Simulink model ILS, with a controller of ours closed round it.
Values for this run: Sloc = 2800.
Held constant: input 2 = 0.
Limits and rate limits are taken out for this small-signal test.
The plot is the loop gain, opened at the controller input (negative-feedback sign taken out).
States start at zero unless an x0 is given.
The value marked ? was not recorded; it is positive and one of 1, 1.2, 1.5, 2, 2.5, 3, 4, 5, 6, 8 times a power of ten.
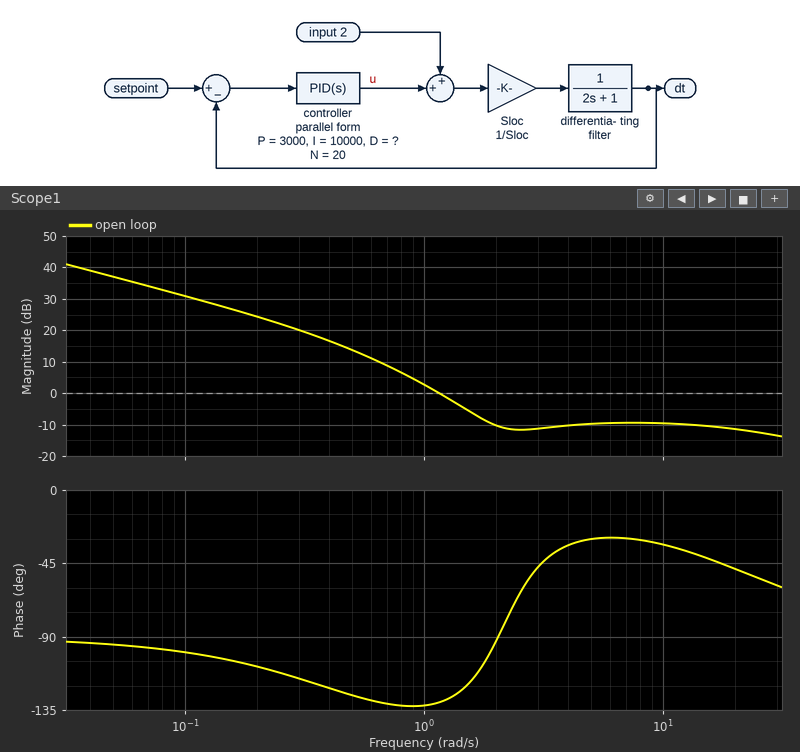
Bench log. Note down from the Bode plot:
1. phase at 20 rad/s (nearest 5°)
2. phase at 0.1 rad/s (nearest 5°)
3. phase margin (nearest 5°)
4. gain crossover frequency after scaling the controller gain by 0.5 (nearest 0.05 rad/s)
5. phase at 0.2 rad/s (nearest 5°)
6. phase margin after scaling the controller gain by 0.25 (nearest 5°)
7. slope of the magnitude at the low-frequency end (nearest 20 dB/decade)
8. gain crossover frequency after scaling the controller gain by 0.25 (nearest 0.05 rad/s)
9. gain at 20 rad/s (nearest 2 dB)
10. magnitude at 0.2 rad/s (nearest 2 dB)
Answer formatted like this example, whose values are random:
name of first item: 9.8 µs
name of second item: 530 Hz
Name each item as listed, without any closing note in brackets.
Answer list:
phase at 20 rad/s: -50°
phase at 0.1 rad/s: -100°
phase margin: 50°
gain crossover frequency after scaling the controller gain by 0.5: 0.85 rad/s
phase at 0.2 rad/s: -110°
phase margin after scaling the controller gain by 0.25: 50°
slope of the magnitude at the low-frequency end: -20 dB/decade
gain crossover frequency after scaling the controller gain by 0.25: 0.55 rad/s
gain at 20 rad/s: -12 dB
magnitude at 0.2 rad/s: 24 dB
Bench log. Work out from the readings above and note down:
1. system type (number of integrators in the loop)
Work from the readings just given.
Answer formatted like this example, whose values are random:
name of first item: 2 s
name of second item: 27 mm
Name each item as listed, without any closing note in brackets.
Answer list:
system type: 1
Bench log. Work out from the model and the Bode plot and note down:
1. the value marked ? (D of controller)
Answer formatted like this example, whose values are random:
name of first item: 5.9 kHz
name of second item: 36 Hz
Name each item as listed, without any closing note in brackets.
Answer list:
the value marked ?: 2000
